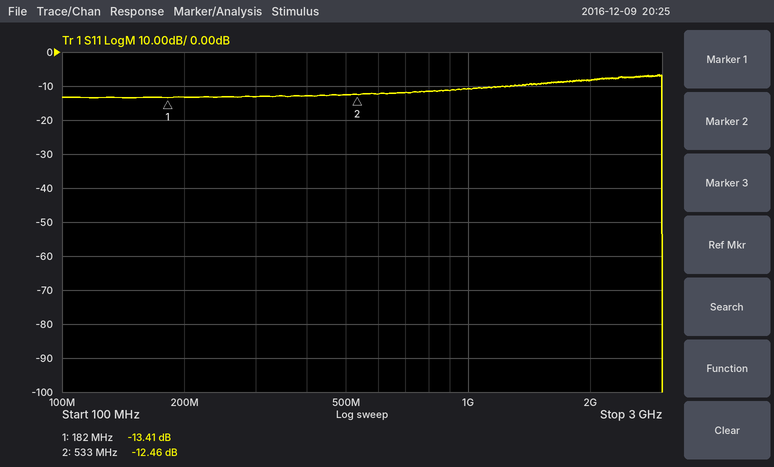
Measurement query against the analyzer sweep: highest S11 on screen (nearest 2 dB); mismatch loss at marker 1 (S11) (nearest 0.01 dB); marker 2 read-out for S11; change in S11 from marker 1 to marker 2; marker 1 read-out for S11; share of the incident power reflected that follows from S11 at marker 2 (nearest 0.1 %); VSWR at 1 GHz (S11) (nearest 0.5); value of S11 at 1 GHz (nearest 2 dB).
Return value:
-6 dB
0.20 dB
-12.46 dB
0.95 dB
-13.41 dB
5.7 %
2.0
-10 dB
